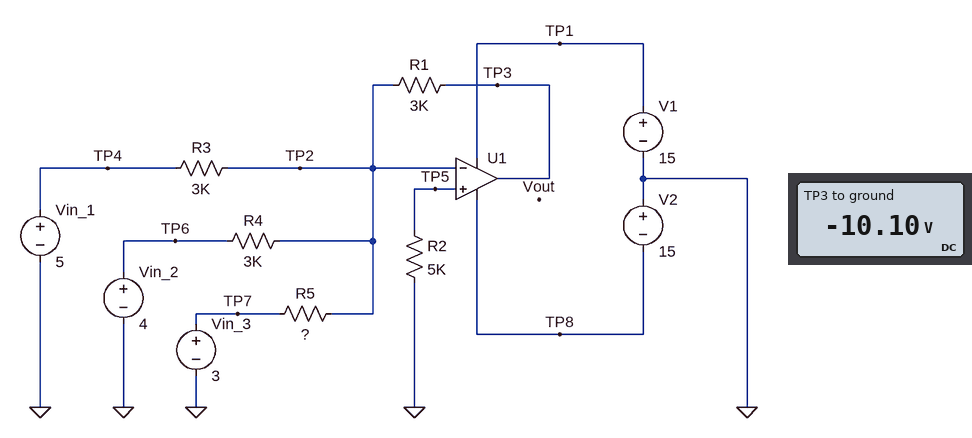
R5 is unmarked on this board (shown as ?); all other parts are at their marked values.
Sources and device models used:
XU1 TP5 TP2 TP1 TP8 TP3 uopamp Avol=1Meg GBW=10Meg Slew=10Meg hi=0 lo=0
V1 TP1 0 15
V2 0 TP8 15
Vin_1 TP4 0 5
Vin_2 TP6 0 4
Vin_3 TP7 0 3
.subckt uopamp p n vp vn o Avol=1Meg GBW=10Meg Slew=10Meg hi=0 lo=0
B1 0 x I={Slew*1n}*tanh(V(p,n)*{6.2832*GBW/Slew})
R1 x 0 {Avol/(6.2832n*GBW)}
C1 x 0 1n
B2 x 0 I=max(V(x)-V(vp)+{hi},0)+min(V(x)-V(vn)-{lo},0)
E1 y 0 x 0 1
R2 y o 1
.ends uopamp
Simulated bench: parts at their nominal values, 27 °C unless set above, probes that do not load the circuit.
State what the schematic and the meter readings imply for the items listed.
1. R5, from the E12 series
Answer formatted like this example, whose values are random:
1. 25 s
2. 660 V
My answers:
1. 8.2 kΩ
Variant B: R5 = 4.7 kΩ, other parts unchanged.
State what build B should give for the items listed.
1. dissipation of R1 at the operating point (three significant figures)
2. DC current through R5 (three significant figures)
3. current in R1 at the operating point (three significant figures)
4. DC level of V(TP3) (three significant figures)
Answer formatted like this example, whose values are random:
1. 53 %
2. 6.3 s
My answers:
1. 39.7 mW
2. 638 µA
3. 3.64 mA
4. -10.9 V
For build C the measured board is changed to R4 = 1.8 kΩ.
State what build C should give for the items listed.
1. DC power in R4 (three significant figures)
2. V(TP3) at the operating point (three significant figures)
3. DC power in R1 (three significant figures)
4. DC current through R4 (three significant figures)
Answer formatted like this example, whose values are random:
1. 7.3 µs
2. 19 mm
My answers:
1. 8.89 mW
2. -12.8 V
3. 54.3 mW
4. 2.22 mA
